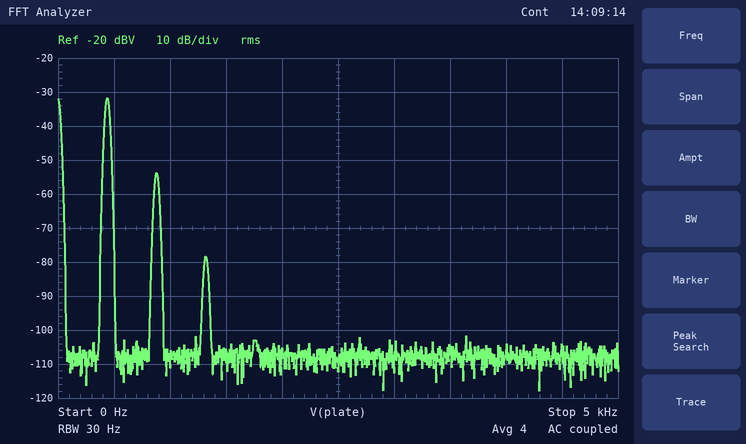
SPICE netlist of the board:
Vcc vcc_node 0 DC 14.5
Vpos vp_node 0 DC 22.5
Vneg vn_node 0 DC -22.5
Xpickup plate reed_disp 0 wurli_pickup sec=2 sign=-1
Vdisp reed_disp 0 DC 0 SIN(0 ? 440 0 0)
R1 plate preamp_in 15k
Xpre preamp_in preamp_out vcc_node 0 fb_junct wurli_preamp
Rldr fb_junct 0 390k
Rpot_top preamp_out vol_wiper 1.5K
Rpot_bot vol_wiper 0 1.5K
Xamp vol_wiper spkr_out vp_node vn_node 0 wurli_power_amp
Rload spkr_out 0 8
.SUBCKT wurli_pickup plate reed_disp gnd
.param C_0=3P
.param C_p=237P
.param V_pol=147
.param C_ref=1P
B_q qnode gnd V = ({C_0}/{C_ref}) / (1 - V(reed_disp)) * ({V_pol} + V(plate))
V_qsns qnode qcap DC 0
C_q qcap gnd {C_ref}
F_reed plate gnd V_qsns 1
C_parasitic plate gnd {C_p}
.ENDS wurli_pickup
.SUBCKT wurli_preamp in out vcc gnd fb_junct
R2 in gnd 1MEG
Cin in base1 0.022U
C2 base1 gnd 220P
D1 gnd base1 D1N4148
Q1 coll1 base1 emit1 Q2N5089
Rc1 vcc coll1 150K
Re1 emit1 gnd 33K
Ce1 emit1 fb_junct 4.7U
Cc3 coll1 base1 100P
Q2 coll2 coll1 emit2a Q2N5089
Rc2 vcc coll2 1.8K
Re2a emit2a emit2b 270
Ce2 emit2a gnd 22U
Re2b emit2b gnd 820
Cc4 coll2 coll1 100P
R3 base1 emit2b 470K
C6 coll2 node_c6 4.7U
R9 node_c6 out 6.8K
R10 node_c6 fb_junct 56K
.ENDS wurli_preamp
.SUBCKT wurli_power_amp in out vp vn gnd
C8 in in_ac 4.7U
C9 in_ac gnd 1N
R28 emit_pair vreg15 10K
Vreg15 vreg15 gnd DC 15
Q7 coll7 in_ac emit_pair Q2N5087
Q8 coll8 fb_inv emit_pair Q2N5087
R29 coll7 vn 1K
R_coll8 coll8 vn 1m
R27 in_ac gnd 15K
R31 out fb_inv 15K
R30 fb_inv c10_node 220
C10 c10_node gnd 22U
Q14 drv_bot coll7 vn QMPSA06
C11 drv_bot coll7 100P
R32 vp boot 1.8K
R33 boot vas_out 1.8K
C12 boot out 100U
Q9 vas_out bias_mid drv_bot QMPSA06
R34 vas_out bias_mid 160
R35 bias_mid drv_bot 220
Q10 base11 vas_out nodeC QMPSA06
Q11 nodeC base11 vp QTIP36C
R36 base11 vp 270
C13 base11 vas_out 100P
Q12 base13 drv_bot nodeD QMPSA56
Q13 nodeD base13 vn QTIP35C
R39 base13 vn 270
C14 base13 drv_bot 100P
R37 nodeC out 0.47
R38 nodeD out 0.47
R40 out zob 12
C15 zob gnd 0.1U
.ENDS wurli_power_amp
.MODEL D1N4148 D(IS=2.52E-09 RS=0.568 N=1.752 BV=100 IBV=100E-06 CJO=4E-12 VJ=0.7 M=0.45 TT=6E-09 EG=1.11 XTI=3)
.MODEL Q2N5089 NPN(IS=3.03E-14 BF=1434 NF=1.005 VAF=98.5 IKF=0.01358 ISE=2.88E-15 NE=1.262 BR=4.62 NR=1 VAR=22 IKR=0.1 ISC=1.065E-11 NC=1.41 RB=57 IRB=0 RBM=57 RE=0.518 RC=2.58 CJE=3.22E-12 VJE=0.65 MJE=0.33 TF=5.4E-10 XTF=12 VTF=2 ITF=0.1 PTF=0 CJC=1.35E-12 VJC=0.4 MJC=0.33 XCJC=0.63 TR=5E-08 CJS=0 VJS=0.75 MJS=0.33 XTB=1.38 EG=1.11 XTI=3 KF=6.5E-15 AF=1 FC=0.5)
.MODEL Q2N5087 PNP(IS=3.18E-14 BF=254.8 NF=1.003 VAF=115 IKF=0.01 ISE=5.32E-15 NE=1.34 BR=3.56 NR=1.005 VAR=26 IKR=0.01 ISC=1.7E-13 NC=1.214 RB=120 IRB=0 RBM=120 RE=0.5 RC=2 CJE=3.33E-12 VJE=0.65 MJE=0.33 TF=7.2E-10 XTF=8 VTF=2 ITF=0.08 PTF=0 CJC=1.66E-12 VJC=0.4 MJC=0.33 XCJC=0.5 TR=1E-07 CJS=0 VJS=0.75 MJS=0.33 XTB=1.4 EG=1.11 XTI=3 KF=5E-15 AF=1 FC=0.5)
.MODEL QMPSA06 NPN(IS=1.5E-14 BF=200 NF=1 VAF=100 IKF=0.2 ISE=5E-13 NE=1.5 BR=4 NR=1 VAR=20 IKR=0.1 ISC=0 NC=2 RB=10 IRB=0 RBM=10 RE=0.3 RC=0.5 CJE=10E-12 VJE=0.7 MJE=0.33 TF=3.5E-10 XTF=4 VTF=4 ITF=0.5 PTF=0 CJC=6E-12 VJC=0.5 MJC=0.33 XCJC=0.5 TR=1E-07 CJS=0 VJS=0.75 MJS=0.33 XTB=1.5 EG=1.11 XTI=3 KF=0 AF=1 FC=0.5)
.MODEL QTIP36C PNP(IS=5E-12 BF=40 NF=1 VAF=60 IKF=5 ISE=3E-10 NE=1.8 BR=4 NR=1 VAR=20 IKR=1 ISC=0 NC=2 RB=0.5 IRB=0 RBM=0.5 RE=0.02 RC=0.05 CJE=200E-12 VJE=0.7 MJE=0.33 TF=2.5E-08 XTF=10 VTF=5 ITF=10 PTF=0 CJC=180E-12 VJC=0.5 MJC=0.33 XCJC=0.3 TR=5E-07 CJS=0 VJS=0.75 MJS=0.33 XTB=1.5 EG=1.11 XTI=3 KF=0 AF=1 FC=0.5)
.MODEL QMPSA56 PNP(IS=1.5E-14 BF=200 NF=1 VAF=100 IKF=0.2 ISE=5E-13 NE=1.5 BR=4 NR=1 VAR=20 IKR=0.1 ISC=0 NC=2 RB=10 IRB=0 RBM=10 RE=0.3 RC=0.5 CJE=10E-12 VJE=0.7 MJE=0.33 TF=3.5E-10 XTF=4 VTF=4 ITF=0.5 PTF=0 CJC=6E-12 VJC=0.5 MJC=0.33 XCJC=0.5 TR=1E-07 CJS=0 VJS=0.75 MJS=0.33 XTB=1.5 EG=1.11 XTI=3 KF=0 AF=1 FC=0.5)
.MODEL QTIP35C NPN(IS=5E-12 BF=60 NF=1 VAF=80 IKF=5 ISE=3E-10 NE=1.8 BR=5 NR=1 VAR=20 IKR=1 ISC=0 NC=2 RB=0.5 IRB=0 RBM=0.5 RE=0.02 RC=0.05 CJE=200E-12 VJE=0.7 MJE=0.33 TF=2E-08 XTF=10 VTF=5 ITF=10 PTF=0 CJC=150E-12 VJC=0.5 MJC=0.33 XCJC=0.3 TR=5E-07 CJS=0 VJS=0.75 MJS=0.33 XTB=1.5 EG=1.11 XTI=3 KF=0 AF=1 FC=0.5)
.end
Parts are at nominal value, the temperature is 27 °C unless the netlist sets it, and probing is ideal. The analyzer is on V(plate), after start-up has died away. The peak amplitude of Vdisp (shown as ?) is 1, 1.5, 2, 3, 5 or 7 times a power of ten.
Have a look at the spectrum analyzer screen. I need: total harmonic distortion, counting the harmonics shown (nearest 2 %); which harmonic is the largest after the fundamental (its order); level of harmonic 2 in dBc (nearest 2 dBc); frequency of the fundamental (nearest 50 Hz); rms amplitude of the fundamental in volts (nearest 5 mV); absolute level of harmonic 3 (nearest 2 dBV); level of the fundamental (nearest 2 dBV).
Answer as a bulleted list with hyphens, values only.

- 8 %
- 2
- -22 dBc
- 450 Hz
- 25 mV
- -78 dBV
- -32 dBV
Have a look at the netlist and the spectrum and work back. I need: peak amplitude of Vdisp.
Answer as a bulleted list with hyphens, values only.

- 100 mV
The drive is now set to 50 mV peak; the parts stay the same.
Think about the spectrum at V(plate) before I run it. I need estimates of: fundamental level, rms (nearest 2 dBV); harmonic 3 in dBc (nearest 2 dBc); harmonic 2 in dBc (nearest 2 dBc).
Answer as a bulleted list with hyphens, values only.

- -38 dBV
- -58 dBc
- -28 dBc
